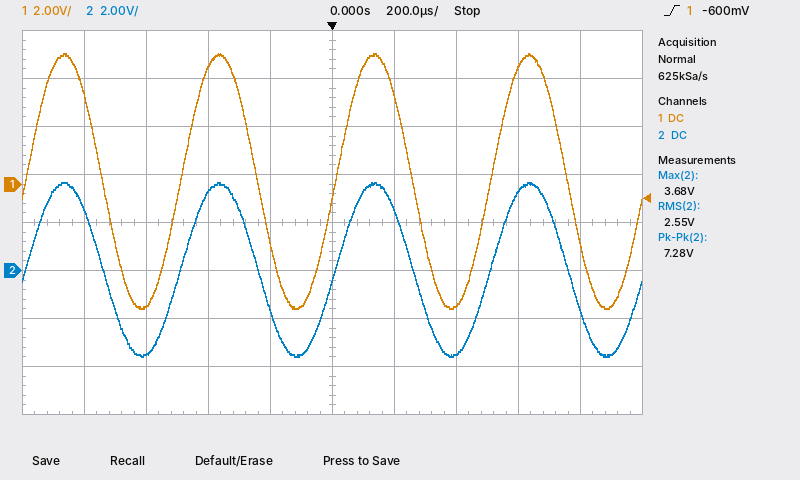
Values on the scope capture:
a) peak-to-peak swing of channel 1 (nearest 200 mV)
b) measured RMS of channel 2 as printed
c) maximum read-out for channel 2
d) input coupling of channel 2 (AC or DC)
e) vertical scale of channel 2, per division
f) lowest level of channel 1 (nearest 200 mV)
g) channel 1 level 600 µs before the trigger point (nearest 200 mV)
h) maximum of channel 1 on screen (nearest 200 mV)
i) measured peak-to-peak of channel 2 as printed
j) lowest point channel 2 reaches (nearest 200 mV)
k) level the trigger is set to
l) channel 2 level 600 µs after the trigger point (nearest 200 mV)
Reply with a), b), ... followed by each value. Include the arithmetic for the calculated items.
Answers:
a) 5.4 V − (-5.2 V) = 10.6 V
b) 2.55 V
c) 3.68 V
d) DC
e) 2 V
f) -5.2 V
g) -5.0 V
h) 5.4 V
i) 7.28 V
j) -3.6 V
k) -600 mV
l) 3.2 V
